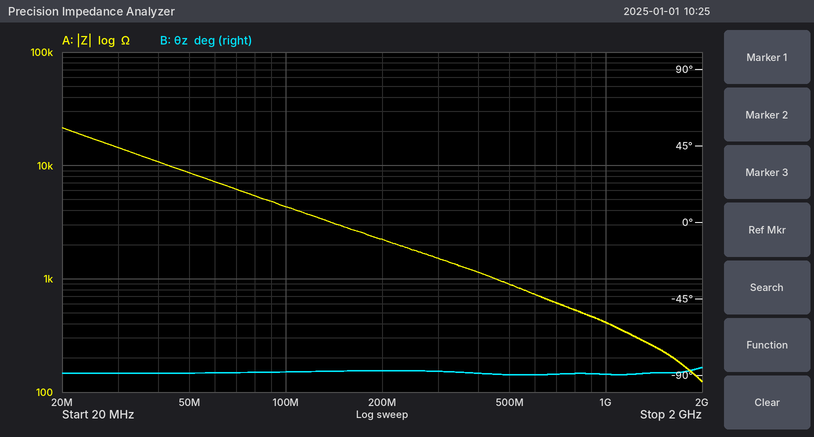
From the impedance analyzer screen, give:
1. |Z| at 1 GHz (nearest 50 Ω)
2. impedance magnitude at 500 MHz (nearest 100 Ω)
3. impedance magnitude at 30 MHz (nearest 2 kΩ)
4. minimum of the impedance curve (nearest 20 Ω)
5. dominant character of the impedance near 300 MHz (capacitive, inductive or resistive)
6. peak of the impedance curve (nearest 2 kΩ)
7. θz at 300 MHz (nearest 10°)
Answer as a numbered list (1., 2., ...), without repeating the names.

1. 400 Ω
2. 900 Ω
3. 14 kΩ
4. 120 Ω
5. capacitive
6. 22 kΩ
7. -90°
